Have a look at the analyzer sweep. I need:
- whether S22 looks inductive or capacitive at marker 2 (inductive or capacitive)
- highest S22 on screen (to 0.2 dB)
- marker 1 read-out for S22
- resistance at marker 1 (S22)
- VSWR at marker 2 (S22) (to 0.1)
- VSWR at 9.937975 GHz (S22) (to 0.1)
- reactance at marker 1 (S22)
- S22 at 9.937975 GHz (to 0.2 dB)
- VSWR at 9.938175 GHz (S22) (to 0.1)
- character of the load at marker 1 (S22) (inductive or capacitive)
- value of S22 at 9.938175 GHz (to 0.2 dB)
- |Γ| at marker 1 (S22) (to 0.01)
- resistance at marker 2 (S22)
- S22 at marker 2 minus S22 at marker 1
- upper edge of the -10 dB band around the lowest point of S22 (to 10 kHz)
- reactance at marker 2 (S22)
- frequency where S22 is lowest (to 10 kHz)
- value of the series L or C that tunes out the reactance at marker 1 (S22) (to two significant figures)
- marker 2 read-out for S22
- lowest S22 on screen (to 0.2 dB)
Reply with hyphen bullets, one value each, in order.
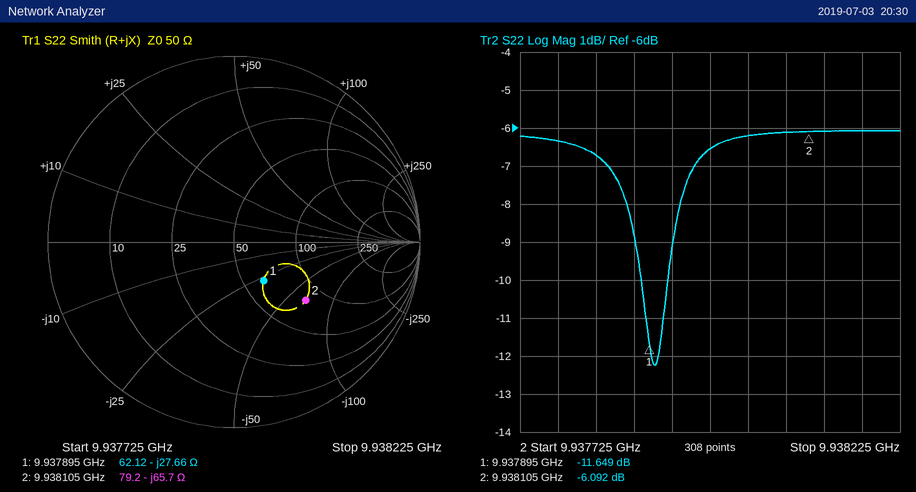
- capacitive
- -6.0 dB
- -11.649 dB
- 62.12 Ω
- 3.0
- 2.8
- -27.66 Ω
- -6.6 dB
- 3.0
- capacitive
- -6.0 dB
- 0.26
- 79.2 Ω
- 5.557 dB
- 9.93792 GHz
- -65.7 Ω
- 9.93790 GHz
- 440 pH
- -6.092 dB
- -12.2 dB
